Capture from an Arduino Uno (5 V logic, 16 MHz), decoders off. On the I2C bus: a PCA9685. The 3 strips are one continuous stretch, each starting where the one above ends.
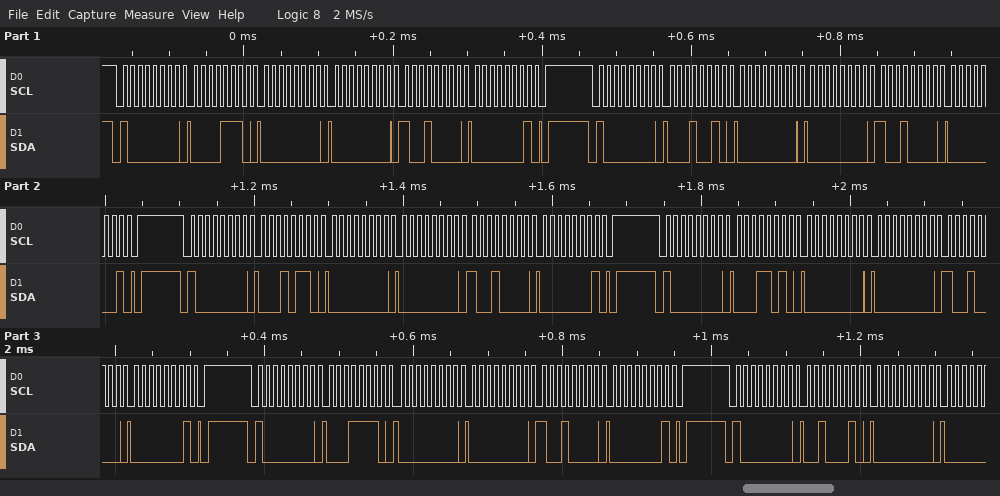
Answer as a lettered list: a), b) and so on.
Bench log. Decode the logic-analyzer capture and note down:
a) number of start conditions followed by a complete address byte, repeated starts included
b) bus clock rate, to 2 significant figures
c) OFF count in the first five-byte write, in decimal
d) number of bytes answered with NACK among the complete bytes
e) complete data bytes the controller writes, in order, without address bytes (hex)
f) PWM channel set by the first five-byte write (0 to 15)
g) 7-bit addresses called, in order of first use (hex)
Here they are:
a) 6
b) 100 kHz
c) 400
d) 0
e) 0E 00 00 90 01 12 00 00 90 01 16 00 00 90 01 1A 00 00 90 01 1E 00 00 90 01 22 00
f) 2
g) 0x40
